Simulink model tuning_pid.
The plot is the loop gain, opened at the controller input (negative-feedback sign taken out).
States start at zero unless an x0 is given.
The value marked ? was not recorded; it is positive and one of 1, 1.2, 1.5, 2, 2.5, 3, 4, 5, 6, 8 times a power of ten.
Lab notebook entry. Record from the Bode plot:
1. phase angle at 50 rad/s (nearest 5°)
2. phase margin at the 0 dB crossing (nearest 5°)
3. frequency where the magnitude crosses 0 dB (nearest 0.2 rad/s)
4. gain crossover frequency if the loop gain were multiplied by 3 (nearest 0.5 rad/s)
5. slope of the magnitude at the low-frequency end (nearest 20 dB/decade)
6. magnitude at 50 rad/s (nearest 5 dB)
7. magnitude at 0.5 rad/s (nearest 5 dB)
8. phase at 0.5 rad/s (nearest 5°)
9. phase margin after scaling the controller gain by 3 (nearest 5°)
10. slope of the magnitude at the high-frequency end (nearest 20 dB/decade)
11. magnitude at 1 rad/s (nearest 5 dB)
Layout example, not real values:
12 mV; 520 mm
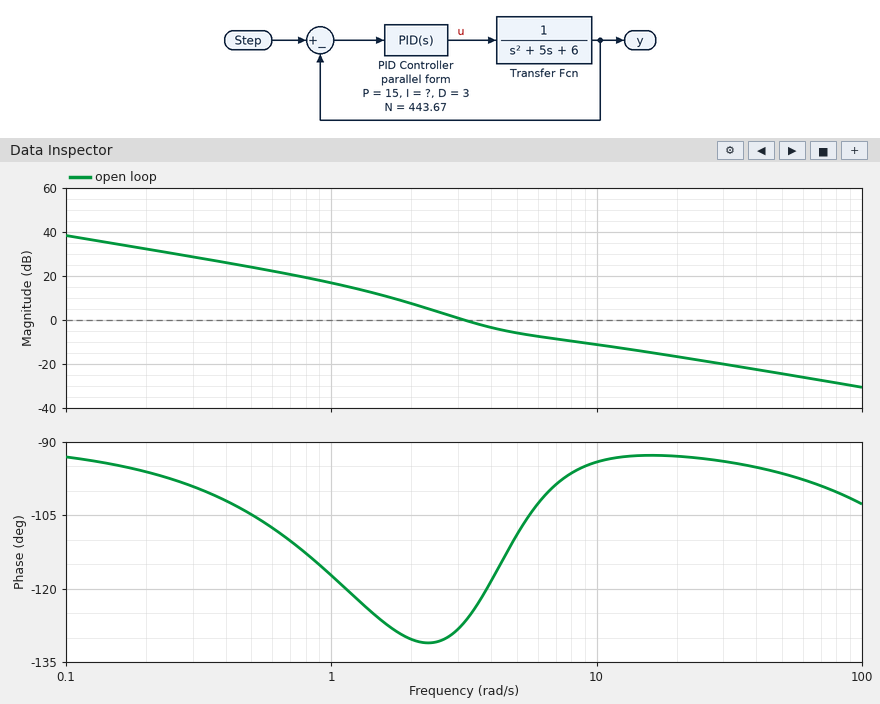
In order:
-95°; 55°; 3.2 rad/s; 8.0 rad/s; -20 dB/decade; -25 dB; 25 dB; -105°; 85°; -20 dB/decade; 15 dB
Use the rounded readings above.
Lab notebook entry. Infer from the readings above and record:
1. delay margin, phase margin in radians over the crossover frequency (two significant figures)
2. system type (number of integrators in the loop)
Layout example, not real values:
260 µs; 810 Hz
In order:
0.30 s; 1
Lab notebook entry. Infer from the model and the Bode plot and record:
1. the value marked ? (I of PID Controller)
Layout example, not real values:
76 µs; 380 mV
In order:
50
